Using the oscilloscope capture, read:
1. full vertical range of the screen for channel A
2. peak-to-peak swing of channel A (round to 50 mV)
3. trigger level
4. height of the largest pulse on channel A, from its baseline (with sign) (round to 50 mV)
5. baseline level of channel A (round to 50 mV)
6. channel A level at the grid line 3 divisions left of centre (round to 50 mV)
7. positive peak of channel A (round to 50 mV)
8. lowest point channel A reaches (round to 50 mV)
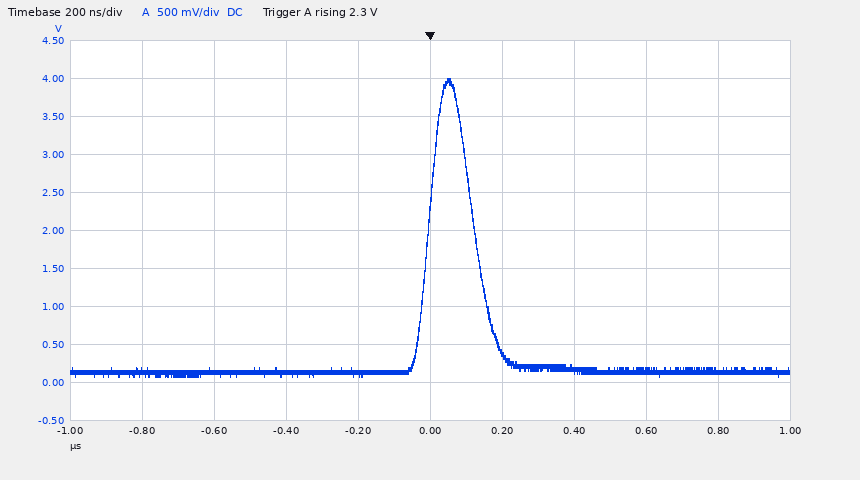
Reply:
5 V
3.90 V
2.3 V
+3.85 V
150 mV
150 mV
4.00 V
100 mV
